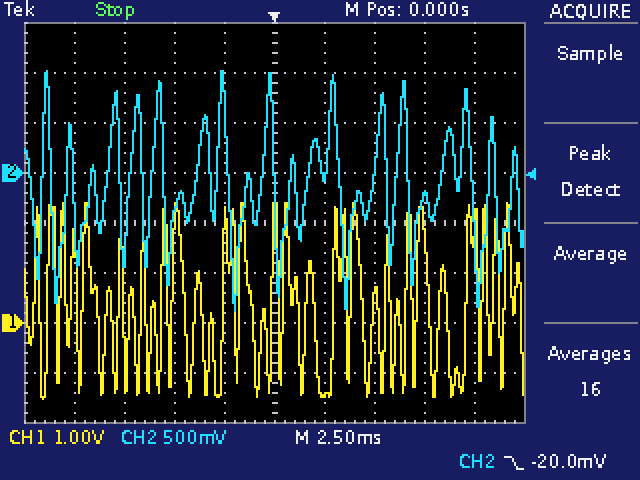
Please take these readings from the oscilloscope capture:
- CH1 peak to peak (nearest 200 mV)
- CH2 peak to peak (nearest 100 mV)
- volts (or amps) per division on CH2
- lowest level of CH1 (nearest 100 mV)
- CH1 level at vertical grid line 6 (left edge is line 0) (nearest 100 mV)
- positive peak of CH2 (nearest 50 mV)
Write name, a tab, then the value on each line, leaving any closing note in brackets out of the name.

CH1 peak to peak	4.0 V
CH2 peak to peak	2.40 V
volts (or amps) per division on CH2	500 mV
lowest level of CH1	-1.5 V
CH1 level at vertical grid line 6 (left edge is line 0)	-1.4 V
positive peak of CH2	1.00 V
